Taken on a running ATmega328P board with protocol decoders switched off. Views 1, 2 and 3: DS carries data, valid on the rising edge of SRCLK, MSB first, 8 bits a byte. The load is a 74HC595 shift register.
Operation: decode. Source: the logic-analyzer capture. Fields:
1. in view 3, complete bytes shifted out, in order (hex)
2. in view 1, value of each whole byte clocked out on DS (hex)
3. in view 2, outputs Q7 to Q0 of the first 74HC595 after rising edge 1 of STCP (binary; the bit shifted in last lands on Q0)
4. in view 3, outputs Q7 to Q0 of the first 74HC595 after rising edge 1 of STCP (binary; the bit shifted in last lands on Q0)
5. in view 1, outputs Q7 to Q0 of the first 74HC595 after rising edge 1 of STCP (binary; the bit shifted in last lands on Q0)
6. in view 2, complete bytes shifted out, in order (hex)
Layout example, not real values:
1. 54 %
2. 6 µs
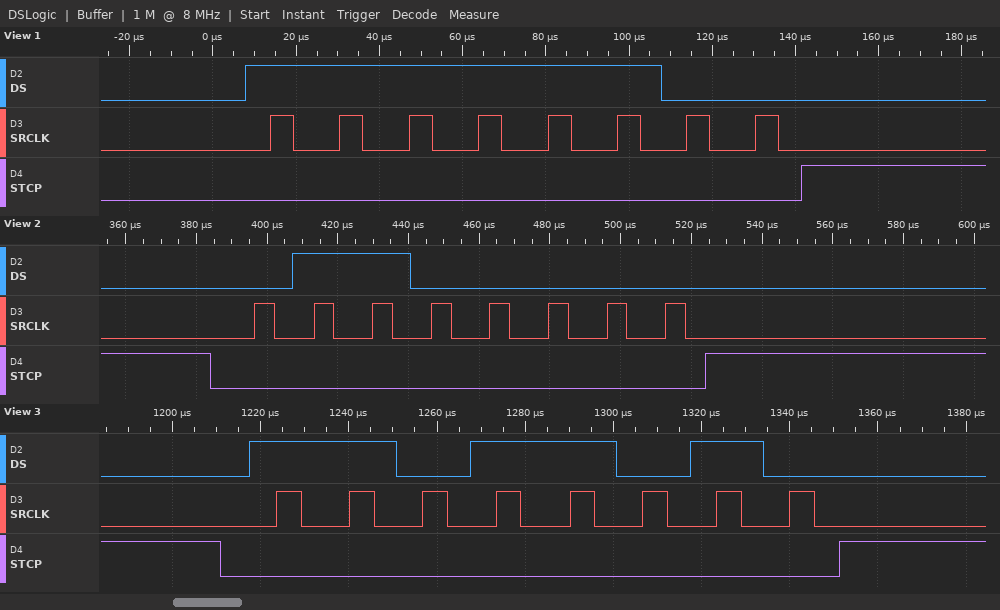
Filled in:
1. DA
2. FC
3. 01100000
4. 11011010
5. 11111100
6. 60
